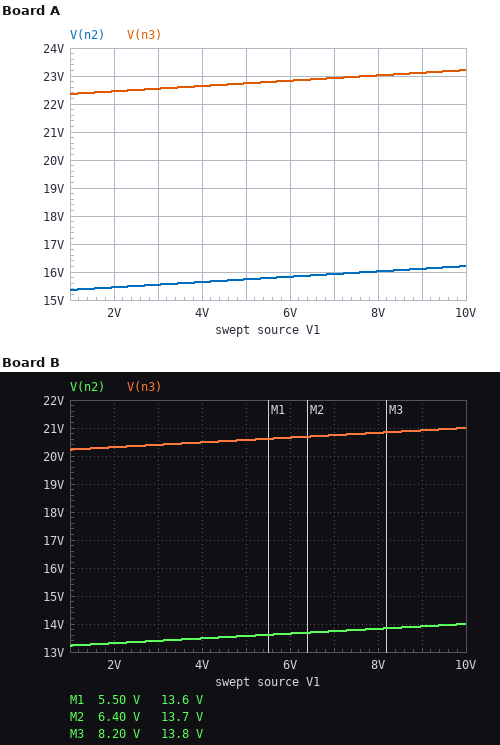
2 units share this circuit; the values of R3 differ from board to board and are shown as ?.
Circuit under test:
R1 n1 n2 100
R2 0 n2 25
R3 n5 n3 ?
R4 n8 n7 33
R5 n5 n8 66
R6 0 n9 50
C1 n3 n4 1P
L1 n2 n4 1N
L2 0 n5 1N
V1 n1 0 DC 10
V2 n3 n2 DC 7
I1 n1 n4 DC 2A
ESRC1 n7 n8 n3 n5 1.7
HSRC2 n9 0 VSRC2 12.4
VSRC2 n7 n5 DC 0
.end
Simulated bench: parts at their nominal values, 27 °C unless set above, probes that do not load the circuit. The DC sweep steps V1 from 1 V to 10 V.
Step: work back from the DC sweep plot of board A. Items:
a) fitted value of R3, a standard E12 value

18 Ω
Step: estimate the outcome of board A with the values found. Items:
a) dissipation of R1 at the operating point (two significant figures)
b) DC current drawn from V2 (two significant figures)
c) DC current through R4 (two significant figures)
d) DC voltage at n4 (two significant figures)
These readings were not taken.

390 mW
1.3 A
1.2 A
16 V
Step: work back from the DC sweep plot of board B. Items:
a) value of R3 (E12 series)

15 Ω
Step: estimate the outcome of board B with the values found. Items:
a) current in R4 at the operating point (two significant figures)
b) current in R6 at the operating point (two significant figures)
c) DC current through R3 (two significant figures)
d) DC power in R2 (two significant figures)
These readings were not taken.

1.1 A
130 mA
1.4 A
7.8 W
